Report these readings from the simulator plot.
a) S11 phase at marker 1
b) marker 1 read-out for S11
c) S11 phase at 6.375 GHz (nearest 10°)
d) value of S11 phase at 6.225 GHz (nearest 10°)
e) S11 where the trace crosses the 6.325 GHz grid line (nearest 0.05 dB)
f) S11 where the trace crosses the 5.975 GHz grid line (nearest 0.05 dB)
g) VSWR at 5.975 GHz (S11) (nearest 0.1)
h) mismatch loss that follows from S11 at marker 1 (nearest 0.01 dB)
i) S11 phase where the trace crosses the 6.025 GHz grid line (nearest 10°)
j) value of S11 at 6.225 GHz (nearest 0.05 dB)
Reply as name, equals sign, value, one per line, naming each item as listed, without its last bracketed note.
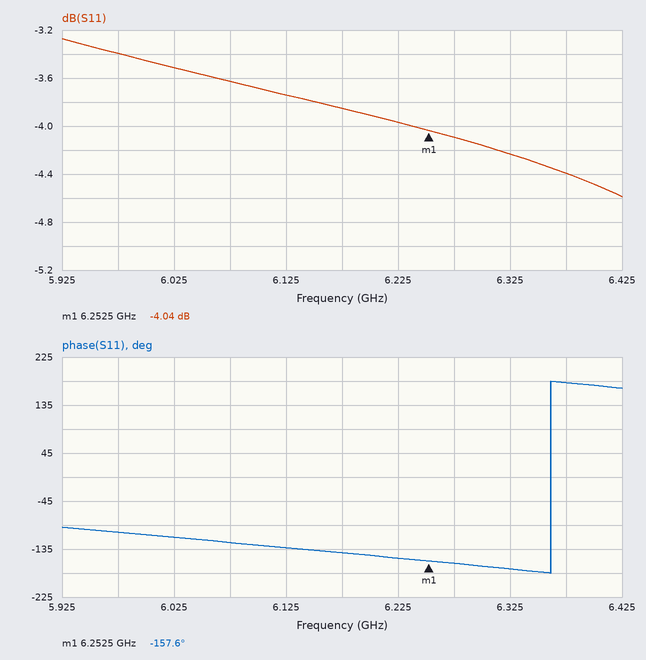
S11 phase at marker 1 = -157.6°
marker 1 read-out for S11 = -4.04 dB
S11 phase at 6.375 GHz = 180°
value of S11 phase at 6.225 GHz = -150°
S11 where the trace crosses the 6.325 GHz grid line = -4.25 dB
S11 where the trace crosses the 5.975 GHz grid line = -3.40 dB
VSWR at 5.975 GHz (S11) = 5.2
mismatch loss that follows from S11 at marker 1 = 2.18 dB
S11 phase where the trace crosses the 6.025 GHz grid line = -110°
value of S11 at 6.225 GHz = -3.95 dB
